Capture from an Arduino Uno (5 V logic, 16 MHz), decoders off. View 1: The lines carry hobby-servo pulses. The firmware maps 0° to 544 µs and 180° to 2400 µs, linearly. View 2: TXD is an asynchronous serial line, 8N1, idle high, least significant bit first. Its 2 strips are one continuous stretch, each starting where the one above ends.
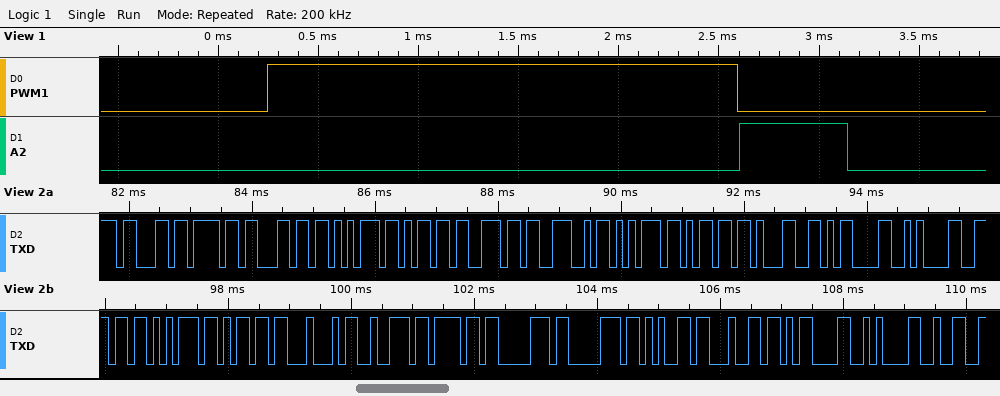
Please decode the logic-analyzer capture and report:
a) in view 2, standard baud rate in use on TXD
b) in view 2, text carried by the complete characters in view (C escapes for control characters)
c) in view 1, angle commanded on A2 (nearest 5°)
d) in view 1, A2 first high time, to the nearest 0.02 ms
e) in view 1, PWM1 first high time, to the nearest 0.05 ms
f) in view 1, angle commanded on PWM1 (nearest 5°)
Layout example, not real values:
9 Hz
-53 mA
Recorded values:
9600 baud
"columnNum1\r\nnumDropped\r\n2"
0°
0.54 ms
2.35 ms
175°
